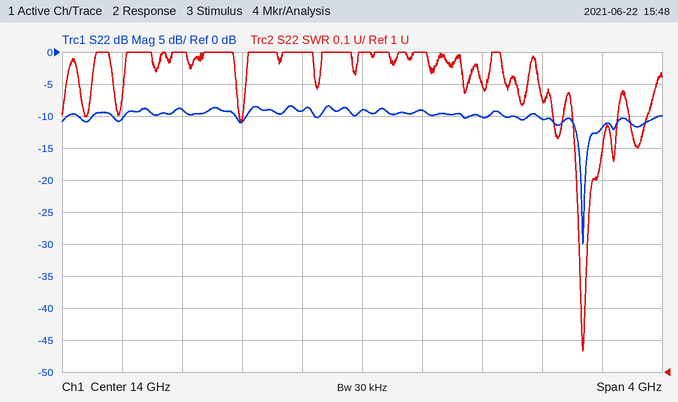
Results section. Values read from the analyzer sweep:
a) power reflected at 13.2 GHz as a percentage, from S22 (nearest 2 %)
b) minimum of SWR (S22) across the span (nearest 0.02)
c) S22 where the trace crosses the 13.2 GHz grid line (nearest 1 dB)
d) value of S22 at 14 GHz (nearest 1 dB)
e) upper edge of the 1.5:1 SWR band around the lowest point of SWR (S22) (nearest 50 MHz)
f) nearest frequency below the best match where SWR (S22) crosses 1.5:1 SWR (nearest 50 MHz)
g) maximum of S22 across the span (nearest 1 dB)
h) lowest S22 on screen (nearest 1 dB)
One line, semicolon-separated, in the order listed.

8 %; 1.06; -11 dB; -9 dB; 15.50 GHz; 15.45 GHz; -8 dB; -30 dB
